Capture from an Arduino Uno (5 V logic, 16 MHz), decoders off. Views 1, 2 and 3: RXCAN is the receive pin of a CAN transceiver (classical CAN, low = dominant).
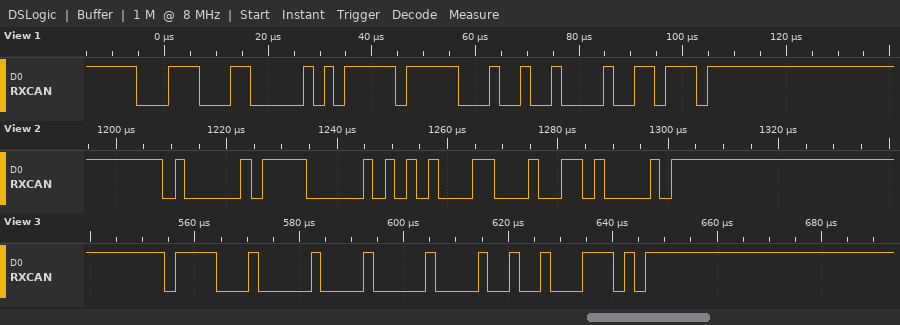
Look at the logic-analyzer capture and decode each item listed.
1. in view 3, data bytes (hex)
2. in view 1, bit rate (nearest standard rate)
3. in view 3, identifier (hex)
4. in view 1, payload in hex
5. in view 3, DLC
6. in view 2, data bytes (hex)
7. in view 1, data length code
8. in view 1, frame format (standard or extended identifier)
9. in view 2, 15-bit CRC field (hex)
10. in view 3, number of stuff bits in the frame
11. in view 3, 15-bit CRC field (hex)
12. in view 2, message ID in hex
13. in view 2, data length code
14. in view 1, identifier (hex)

00
500 kbit/s
0x788
FF C9
1
51
2
standard
0x44D0
2
0x248E
0x40F
1
0x1C6
